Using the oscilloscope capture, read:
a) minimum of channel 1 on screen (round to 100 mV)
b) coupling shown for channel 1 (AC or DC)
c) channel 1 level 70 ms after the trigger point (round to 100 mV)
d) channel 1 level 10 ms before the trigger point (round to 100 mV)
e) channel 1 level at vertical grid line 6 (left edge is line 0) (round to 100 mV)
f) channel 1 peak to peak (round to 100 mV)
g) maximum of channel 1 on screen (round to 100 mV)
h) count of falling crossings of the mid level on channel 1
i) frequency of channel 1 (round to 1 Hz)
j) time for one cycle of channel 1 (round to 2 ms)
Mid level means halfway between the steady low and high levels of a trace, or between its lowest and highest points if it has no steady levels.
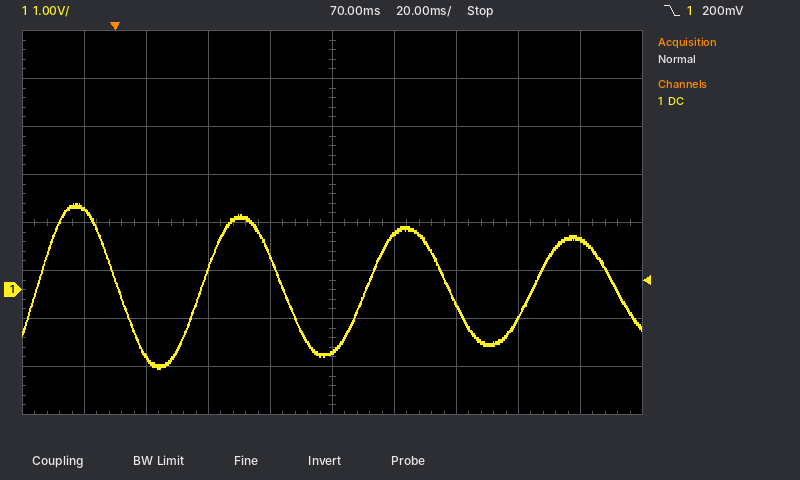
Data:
-1.6 V
DC
-1.3 V
1.7 V
1.2 V
3.4 V
1.8 V
4
19 Hz
54 ms
